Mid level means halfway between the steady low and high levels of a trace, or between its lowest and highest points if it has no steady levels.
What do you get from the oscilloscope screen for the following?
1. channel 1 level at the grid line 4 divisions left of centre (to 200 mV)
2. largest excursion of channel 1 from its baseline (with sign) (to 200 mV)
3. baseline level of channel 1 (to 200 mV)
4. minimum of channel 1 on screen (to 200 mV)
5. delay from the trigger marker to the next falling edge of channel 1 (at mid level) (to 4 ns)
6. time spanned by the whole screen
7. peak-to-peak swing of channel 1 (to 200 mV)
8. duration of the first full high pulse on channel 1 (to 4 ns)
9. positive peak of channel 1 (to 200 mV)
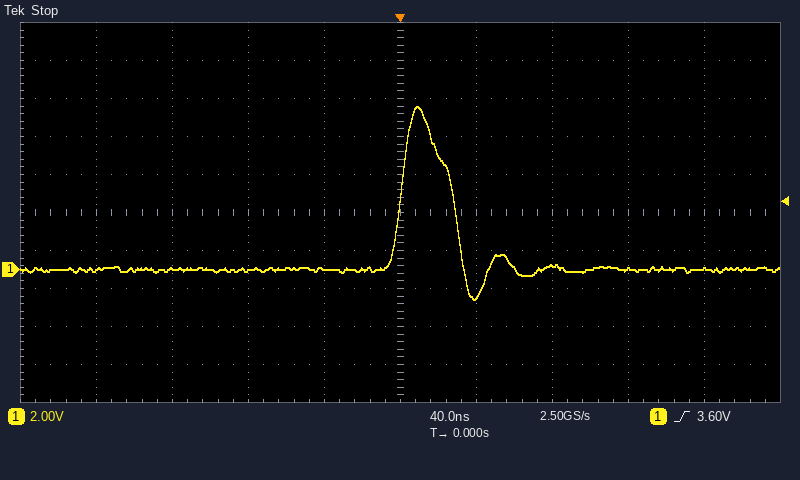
0.0 V
+8.6 V
0.0 V
-1.6 V
28 ns
400 ns
10.2 V
28 ns
8.6 V
